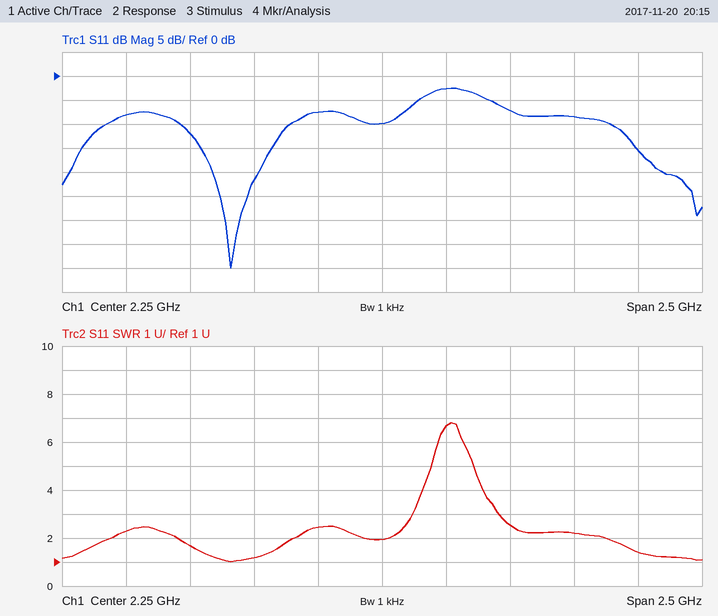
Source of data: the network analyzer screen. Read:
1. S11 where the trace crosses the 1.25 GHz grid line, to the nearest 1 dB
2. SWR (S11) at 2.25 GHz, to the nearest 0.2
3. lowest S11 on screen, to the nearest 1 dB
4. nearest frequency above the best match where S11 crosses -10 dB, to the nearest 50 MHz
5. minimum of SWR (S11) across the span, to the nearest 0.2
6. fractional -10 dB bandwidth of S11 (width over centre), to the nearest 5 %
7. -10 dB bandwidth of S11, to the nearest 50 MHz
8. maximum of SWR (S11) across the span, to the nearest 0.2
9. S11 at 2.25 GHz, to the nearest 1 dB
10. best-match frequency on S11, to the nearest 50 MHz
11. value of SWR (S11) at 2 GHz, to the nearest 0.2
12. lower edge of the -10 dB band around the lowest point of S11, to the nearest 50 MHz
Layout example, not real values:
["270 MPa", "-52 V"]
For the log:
["-8 dB", "2.0", "-40 dB", "1.90 GHz", "1.0", "25 %", "450 MHz", "6.8", "-10 dB", "1.65 GHz", "2.4", "1.45 GHz"]
